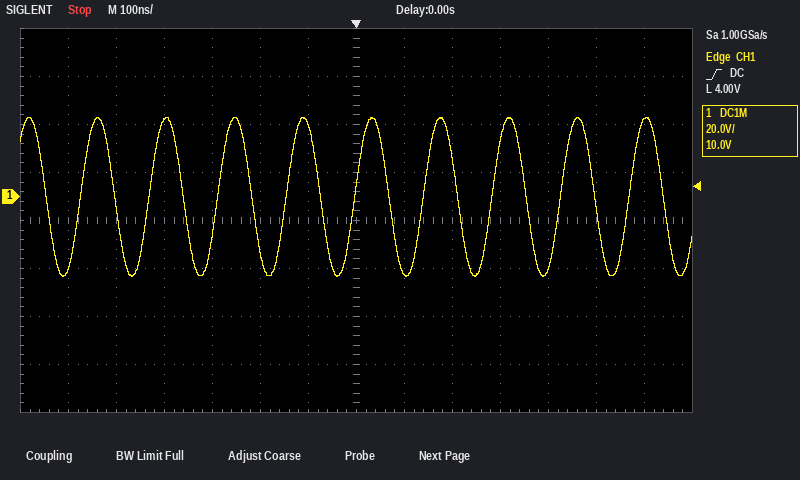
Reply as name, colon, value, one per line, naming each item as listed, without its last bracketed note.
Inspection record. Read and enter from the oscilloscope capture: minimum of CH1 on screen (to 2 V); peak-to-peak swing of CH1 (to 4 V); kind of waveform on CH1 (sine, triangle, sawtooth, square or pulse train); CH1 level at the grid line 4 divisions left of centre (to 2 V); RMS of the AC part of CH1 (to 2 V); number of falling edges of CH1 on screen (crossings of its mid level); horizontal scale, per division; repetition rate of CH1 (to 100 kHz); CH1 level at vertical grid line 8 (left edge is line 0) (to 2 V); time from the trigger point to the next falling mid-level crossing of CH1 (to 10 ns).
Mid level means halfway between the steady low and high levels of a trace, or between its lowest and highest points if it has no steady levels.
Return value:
minimum of CH1 on screen: -34 V
peak-to-peak swing of CH1: 68 V
kind of waveform on CH1: sine
CH1 level at the grid line 4 divisions left of centre: 32 V
RMS of the AC part of CH1: 24 V
number of falling edges of CH1 on screen: 10
horizontal scale, per division: 100 ns
repetition rate of CH1: 7.0 MHz
CH1 level at vertical grid line 8 (left edge is line 0): -32 V
time from the trigger point to the next falling mid-level crossing of CH1: 70 ns
